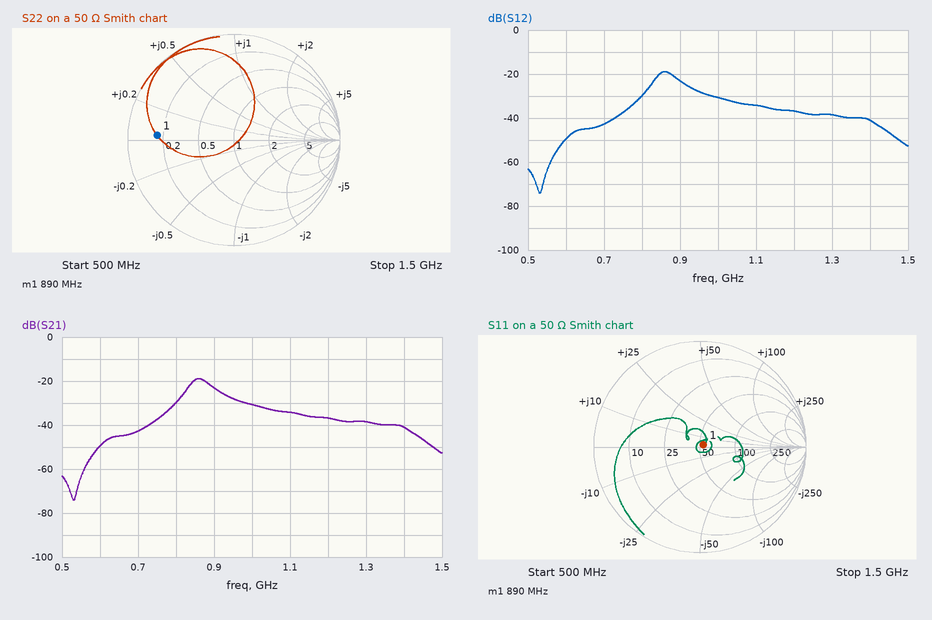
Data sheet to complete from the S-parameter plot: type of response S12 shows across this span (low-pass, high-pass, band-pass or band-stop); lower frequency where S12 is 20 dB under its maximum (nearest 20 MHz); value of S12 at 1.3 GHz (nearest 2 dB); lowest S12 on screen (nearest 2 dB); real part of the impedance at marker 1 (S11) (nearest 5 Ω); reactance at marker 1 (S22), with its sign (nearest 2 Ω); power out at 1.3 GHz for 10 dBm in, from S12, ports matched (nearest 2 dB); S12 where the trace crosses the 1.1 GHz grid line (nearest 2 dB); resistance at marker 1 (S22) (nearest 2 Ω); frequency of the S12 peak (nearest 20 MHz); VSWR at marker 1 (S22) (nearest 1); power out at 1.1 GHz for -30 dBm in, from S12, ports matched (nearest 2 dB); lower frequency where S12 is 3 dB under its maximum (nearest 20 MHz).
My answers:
band-pass
740 MHz
-38 dB
-74 dB
55 Ω
+2 Ω
-28 dBm
-34 dB
8 Ω
860 MHz
6
-64 dBm
840 MHz
